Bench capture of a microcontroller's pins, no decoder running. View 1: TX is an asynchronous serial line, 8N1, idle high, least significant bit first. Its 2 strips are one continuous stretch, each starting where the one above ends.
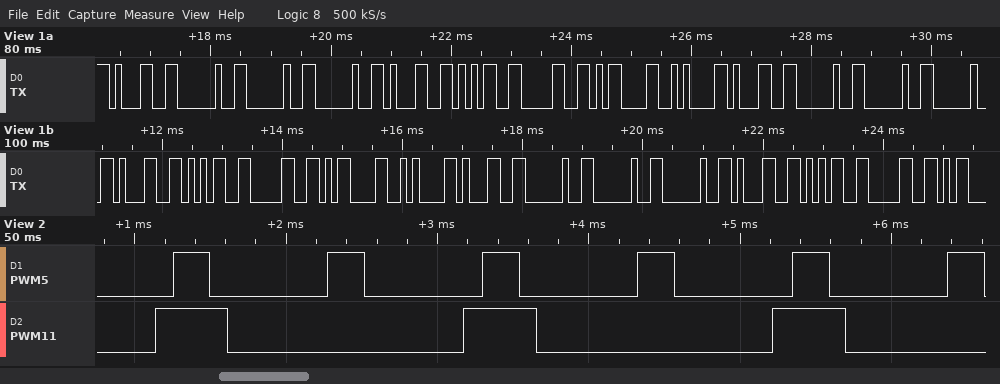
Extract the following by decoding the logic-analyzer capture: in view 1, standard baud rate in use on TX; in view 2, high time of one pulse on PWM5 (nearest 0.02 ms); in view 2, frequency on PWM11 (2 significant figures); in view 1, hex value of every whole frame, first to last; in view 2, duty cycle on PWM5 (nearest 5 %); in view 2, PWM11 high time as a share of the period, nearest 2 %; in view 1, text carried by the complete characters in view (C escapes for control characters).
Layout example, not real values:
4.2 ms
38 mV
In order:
9600 baud
0.24 ms
490 Hz
31 20 20 20 31 35 30 0D 0A 31 20 20 20 31 35 30 0D 0A 31 20 20 20 31 35 30
25 %
24 %
"1   150\r\n1   150\r\n1   150"
